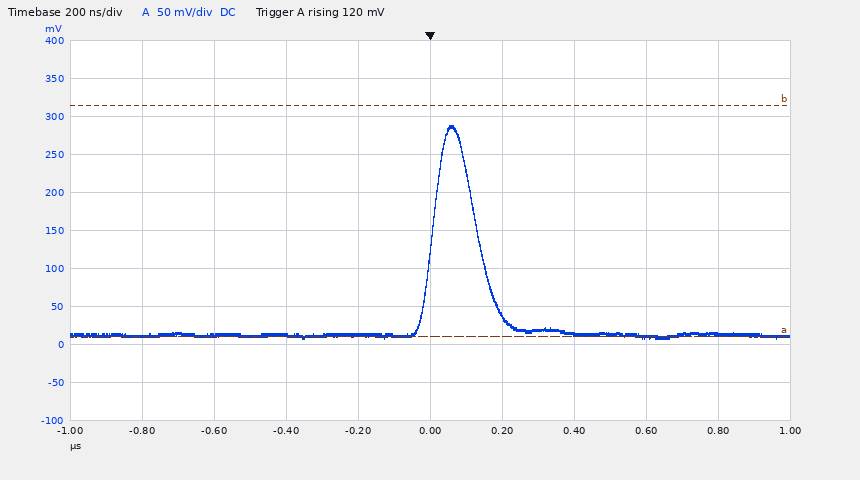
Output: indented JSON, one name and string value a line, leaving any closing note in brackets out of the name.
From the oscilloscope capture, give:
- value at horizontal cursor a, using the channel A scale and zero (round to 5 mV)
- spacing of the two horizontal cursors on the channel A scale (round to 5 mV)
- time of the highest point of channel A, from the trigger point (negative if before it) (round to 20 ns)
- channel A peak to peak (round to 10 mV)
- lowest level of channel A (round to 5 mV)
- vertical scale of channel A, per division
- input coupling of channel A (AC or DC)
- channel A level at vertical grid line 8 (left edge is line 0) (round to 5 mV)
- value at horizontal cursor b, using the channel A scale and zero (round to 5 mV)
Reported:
{
  "value at horizontal cursor a, using the channel A scale and zero": "10 mV",
  "spacing of the two horizontal cursors on the channel A scale": "305 mV",
  "time of the highest point of channel A, from the trigger point (negative if before it)": "+60 ns",
  "channel A peak to peak": "280 mV",
  "lowest level of channel A": "10 mV",
  "vertical scale of channel A, per division": "50 mV",
  "input coupling of channel A": "DC",
  "channel A level at vertical grid line 8 (left edge is line 0)": "10 mV",
  "value at horizontal cursor b, using the channel A scale and zero": "315 mV"
}
